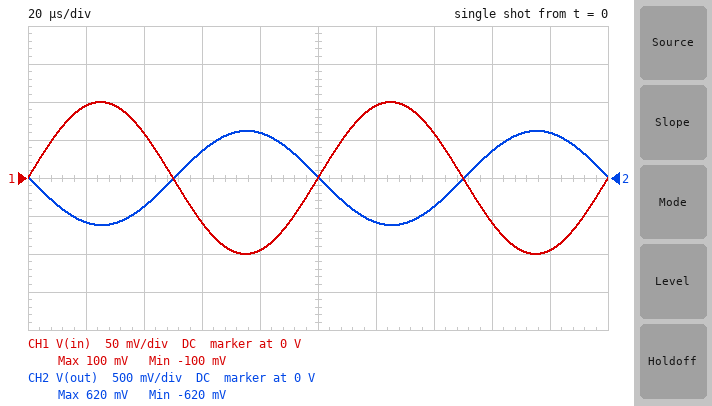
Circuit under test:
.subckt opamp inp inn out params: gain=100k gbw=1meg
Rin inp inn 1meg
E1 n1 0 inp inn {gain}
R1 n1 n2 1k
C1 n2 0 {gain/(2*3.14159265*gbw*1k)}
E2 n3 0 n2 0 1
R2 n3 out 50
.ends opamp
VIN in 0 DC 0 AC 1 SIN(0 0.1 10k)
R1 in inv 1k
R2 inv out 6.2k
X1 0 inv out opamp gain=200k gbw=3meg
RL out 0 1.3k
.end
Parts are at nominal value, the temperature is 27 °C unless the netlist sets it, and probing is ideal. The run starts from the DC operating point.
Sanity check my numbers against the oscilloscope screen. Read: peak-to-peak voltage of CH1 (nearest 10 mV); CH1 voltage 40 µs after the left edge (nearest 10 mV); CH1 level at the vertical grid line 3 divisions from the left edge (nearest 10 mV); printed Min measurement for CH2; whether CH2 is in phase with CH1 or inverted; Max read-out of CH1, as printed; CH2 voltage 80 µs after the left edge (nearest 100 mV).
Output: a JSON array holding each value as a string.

["200 mV", "60 mV", "-60 mV", "-620 mV", "inverted", "100 mV", "600 mV"]
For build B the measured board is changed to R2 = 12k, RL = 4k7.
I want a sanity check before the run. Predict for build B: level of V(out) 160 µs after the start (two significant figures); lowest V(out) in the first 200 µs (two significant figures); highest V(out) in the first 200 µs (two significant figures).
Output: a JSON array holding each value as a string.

["660 mV", "-1.2 V", "1.2 V"]
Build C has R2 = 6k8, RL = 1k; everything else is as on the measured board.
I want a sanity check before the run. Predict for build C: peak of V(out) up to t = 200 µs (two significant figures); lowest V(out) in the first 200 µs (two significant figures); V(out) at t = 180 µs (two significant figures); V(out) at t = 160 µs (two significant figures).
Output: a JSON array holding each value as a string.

["680 mV", "-680 mV", "650 mV", "380 mV"]
